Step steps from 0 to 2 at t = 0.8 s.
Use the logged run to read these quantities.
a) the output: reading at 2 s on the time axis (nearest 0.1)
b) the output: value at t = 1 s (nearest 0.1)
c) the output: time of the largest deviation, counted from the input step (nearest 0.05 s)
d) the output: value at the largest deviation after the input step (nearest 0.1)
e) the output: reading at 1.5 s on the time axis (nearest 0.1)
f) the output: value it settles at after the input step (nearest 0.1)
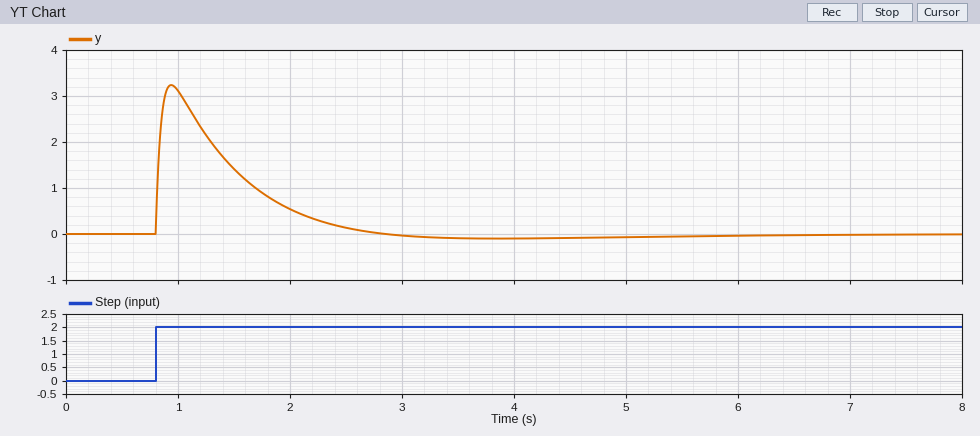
0.5
3.1
0.15 s
3.2
1.4
0.0
